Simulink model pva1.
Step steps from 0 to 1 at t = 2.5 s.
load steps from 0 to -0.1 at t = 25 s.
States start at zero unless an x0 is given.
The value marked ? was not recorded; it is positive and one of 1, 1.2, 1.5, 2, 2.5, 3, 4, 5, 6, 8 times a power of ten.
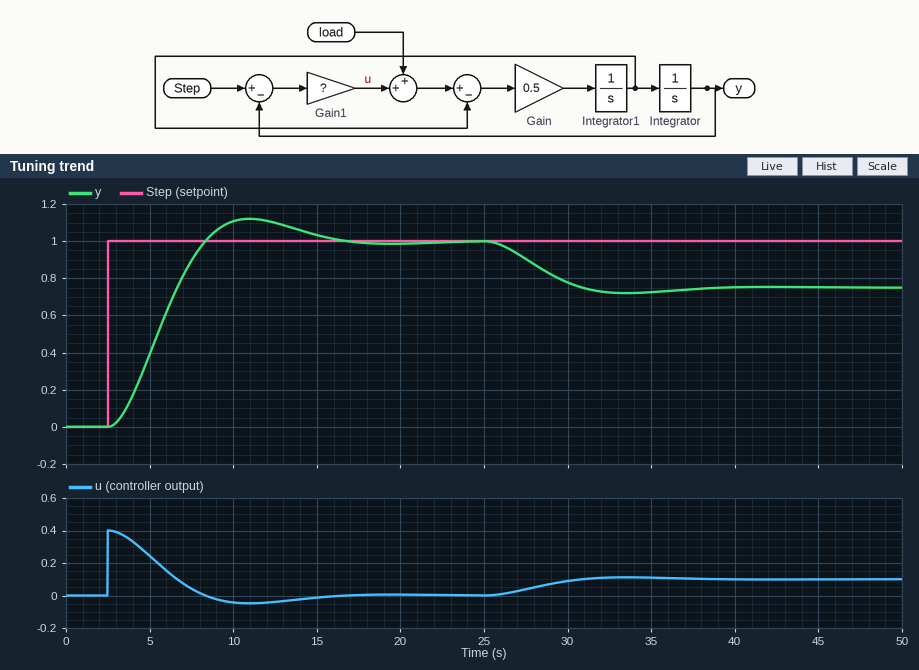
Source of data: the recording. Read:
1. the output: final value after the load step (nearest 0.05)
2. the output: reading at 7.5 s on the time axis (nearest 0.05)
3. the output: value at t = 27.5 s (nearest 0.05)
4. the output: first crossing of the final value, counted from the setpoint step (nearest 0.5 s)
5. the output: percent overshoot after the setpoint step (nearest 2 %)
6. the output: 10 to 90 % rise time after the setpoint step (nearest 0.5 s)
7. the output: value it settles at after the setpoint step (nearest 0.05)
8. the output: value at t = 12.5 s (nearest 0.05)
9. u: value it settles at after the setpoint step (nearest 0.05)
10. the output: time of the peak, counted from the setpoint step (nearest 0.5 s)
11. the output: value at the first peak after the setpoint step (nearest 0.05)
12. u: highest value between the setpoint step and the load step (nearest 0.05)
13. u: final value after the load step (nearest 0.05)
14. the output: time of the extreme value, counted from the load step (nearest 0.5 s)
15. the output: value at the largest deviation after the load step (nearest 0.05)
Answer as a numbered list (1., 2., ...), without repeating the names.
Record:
1. 0.75
2. 0.90
3. 0.90
4. 6.0 s
5. 12 %
6. 4.0 s
7. 1.00
8. 1.10
9. 0.00
10. 8.5 s
11. 1.10
12. 0.40
13. 0.10
14. 8.5 s
15. 0.70
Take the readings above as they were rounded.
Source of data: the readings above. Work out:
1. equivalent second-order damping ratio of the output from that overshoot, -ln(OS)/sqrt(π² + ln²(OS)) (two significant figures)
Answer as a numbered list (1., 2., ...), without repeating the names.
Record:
1. 0.56
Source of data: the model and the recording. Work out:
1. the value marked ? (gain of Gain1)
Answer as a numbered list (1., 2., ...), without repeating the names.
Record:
1. 0.4
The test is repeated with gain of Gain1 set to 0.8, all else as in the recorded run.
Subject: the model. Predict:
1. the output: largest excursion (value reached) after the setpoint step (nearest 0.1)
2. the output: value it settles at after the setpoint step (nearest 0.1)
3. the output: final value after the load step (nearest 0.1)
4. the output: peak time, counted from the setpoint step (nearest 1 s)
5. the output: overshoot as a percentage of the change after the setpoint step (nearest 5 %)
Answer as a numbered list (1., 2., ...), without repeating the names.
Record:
1. 1.3
2. 1.0
3. 0.9
4. 5 s
5. 25 %
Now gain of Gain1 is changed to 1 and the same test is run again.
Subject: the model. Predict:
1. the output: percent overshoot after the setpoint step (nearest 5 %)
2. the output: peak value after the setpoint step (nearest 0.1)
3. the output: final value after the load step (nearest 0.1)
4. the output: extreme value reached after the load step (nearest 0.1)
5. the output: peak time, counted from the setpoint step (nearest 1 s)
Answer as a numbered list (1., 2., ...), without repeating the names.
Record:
1. 30 %
2. 1.3
3. 0.9
4. 0.9
5. 5 s
